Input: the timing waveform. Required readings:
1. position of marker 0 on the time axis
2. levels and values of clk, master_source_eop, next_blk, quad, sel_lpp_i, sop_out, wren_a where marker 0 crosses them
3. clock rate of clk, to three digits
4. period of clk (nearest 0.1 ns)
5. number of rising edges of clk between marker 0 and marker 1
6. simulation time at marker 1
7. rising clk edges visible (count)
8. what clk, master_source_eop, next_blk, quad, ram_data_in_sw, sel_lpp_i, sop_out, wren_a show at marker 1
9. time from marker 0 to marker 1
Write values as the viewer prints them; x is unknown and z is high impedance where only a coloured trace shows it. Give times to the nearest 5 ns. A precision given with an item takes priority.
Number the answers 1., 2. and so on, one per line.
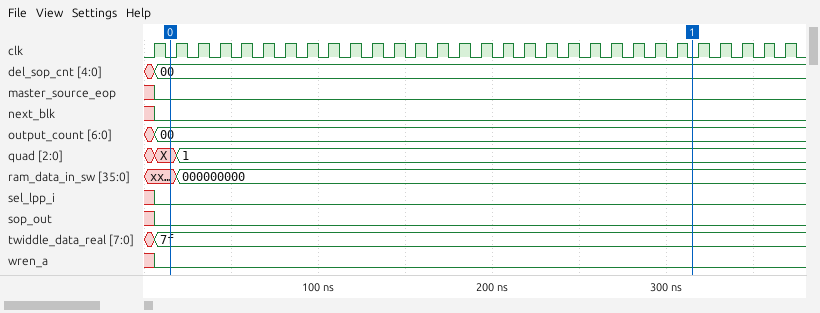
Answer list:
1. 15 ns
2. clk=0, master_source_eop=0, next_blk=0, quad=X, sel_lpp_i=0, sop_out=0, wren_a=0
3. 80.0 MHz
4. 12.5 ns
5. 24
6. 315 ns
7. 30
8. clk=0, master_source_eop=0, next_blk=0, quad=1, ram_data_in_sw=000000000, sel_lpp_i=0, sop_out=0, wren_a=0
9. 300 ns
